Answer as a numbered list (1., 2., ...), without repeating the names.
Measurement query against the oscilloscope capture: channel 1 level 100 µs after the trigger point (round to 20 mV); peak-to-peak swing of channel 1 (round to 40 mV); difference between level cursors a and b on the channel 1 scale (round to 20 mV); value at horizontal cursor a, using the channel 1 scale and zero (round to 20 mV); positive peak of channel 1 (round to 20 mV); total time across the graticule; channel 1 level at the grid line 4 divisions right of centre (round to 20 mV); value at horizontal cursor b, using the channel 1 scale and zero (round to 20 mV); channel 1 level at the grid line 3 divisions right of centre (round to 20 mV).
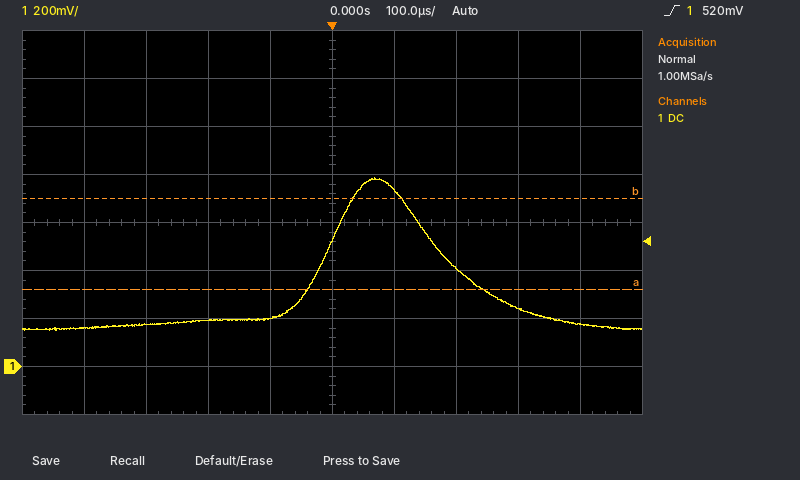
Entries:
1. 740 mV
2. 640 mV
3. 380 mV
4. 320 mV
5. 780 mV
6. 1 ms
7. 180 mV
8. 700 mV
9. 240 mV
